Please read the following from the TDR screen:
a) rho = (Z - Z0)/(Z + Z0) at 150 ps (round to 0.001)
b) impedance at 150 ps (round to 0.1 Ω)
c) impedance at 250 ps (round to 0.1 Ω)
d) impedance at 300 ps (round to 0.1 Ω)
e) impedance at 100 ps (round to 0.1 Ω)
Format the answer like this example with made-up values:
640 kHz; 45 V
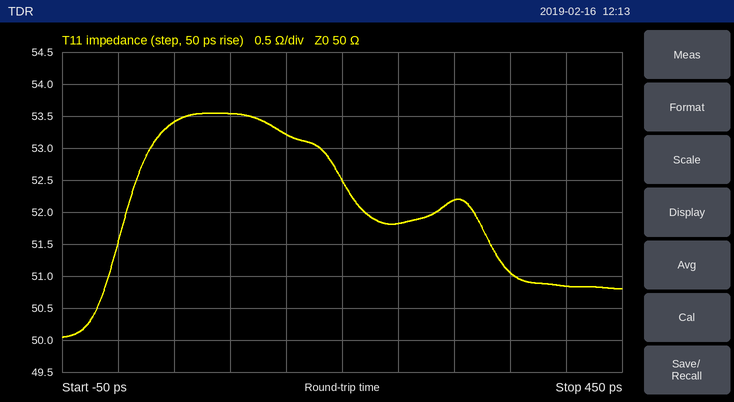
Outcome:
+0.031; 53.2 Ω; 51.8 Ω; 52.2 Ω; 53.5 Ω
